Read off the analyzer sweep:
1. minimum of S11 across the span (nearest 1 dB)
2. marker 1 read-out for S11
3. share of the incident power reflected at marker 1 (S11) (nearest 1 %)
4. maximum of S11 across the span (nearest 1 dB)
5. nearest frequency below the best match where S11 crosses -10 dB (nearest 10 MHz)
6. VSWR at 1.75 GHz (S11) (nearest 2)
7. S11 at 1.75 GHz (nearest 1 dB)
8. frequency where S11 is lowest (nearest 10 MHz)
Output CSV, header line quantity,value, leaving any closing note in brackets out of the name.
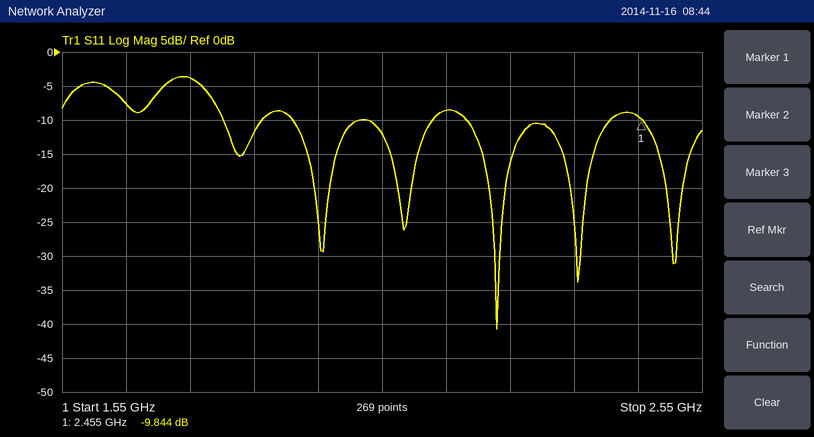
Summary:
quantity,value
minimum of S11 across the span,-41 dB
marker 1 read-out for S11,-9.844 dB
share of the incident power reflected at marker 1 (S11),10 %
maximum of S11 across the span,-4 dB
nearest frequency below the best match where S11 crosses -10 dB,2.18 GHz
VSWR at 1.75 GHz (S11),4
S11 at 1.75 GHz,-4 dB
frequency where S11 is lowest,2.23 GHz
